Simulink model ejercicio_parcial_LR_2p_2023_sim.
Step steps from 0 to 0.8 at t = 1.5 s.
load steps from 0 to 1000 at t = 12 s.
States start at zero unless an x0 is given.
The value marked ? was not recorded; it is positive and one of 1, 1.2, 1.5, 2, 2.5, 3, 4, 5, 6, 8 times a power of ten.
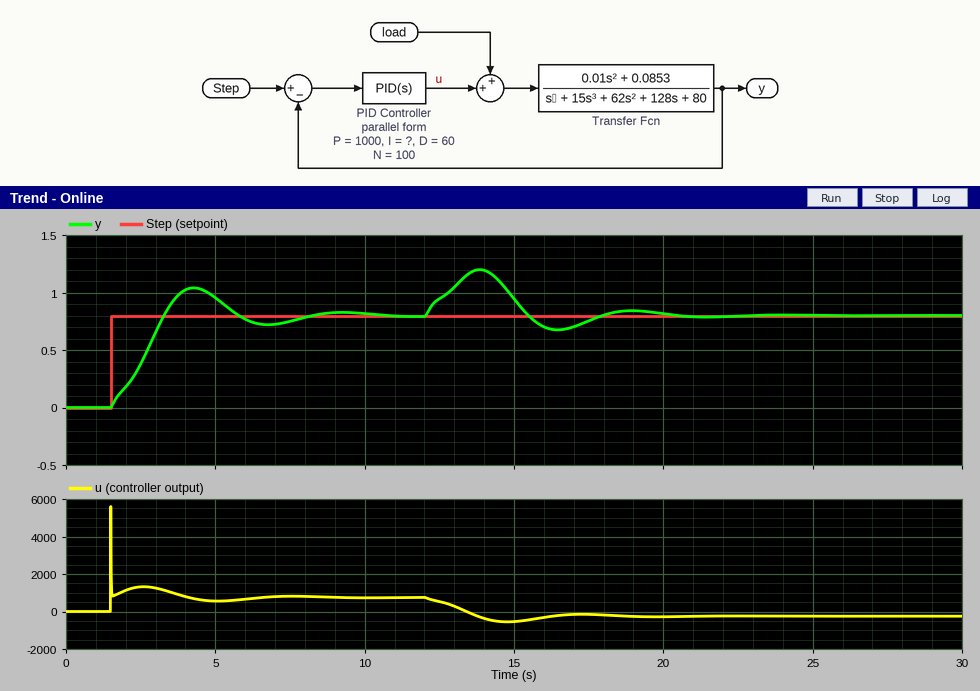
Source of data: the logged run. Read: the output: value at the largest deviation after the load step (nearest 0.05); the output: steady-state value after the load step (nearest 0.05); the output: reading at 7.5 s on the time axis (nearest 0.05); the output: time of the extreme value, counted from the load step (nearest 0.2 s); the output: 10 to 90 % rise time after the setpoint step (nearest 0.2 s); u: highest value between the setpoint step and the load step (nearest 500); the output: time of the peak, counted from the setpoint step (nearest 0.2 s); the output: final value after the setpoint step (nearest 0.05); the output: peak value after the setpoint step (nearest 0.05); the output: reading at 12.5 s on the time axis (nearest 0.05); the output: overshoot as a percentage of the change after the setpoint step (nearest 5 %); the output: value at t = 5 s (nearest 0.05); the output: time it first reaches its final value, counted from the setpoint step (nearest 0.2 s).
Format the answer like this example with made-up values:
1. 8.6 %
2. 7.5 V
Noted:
1. 1.20
2. 0.80
3. 0.75
4. 1.8 s
5. 1.4 s
6. 5500
7. 2.8 s
8. 0.80
9. 1.05
10. 0.95
11. 30 %
12. 0.95
13. 1.8 s
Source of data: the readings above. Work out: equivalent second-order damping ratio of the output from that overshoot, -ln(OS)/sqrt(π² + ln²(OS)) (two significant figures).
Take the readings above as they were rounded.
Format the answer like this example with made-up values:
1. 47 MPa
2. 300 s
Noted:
1. 0.36
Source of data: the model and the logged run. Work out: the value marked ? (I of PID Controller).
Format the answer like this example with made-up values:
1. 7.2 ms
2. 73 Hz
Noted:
1. 1500
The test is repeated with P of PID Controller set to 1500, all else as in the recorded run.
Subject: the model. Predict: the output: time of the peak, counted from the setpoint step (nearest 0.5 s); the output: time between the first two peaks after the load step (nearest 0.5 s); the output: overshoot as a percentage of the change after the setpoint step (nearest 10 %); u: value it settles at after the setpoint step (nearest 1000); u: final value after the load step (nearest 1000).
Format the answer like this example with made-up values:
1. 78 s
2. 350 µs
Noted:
1. 2.5 s
2. 4.5 s
3. 20 %
4. 1000
5. 0
